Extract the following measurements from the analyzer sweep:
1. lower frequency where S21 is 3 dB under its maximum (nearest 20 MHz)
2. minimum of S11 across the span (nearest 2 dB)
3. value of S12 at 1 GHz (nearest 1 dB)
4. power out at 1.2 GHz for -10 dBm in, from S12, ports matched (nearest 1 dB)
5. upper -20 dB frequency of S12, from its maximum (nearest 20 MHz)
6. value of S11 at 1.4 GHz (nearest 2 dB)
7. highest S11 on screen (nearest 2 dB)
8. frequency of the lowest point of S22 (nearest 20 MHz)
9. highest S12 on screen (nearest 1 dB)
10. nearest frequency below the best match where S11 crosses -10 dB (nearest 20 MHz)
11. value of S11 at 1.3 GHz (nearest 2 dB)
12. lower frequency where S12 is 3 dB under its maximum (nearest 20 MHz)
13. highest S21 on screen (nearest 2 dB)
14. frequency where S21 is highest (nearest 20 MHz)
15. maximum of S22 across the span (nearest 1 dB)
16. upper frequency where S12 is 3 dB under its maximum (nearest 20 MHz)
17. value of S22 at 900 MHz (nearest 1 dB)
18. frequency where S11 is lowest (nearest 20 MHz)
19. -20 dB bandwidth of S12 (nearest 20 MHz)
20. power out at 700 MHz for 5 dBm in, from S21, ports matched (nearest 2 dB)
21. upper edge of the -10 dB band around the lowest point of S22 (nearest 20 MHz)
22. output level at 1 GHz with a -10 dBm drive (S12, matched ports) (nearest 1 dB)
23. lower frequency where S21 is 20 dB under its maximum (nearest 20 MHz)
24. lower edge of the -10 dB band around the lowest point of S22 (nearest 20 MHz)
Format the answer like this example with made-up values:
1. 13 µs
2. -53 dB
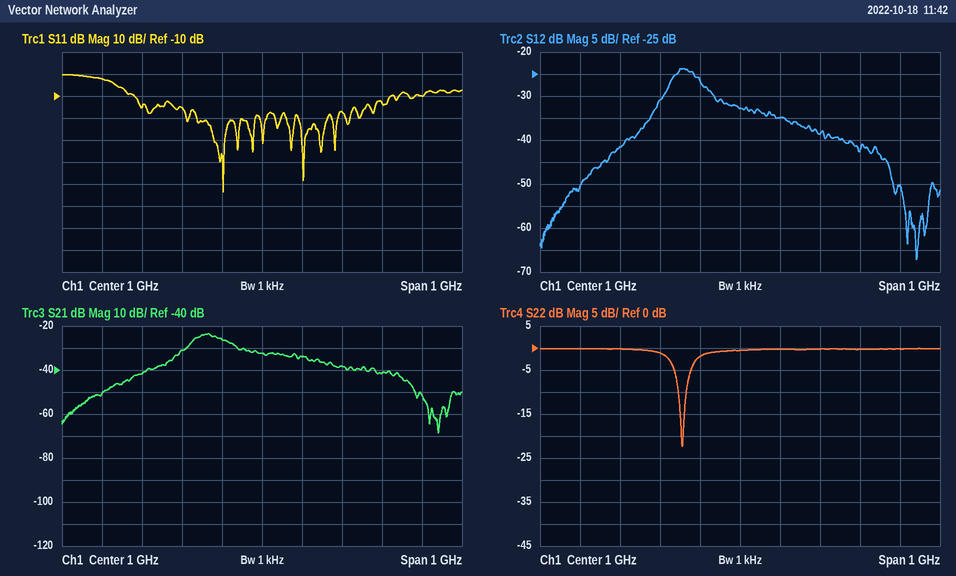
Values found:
1. 820 MHz
2. -54 dB
3. -33 dB
4. -49 dBm
5. 1.36 GHz
6. -10 dB
7. 0 dB
8. 860 MHz
9. -24 dB
10. 680 MHz
11. -14 dB
12. 820 MHz
13. -24 dB
14. 860 MHz
15. 0 dB
16. 900 MHz
17. -2 dB
18. 900 MHz
19. 680 MHz
20. -36 dBm
21. 860 MHz
22. -43 dBm
23. 680 MHz
24. 840 MHz
